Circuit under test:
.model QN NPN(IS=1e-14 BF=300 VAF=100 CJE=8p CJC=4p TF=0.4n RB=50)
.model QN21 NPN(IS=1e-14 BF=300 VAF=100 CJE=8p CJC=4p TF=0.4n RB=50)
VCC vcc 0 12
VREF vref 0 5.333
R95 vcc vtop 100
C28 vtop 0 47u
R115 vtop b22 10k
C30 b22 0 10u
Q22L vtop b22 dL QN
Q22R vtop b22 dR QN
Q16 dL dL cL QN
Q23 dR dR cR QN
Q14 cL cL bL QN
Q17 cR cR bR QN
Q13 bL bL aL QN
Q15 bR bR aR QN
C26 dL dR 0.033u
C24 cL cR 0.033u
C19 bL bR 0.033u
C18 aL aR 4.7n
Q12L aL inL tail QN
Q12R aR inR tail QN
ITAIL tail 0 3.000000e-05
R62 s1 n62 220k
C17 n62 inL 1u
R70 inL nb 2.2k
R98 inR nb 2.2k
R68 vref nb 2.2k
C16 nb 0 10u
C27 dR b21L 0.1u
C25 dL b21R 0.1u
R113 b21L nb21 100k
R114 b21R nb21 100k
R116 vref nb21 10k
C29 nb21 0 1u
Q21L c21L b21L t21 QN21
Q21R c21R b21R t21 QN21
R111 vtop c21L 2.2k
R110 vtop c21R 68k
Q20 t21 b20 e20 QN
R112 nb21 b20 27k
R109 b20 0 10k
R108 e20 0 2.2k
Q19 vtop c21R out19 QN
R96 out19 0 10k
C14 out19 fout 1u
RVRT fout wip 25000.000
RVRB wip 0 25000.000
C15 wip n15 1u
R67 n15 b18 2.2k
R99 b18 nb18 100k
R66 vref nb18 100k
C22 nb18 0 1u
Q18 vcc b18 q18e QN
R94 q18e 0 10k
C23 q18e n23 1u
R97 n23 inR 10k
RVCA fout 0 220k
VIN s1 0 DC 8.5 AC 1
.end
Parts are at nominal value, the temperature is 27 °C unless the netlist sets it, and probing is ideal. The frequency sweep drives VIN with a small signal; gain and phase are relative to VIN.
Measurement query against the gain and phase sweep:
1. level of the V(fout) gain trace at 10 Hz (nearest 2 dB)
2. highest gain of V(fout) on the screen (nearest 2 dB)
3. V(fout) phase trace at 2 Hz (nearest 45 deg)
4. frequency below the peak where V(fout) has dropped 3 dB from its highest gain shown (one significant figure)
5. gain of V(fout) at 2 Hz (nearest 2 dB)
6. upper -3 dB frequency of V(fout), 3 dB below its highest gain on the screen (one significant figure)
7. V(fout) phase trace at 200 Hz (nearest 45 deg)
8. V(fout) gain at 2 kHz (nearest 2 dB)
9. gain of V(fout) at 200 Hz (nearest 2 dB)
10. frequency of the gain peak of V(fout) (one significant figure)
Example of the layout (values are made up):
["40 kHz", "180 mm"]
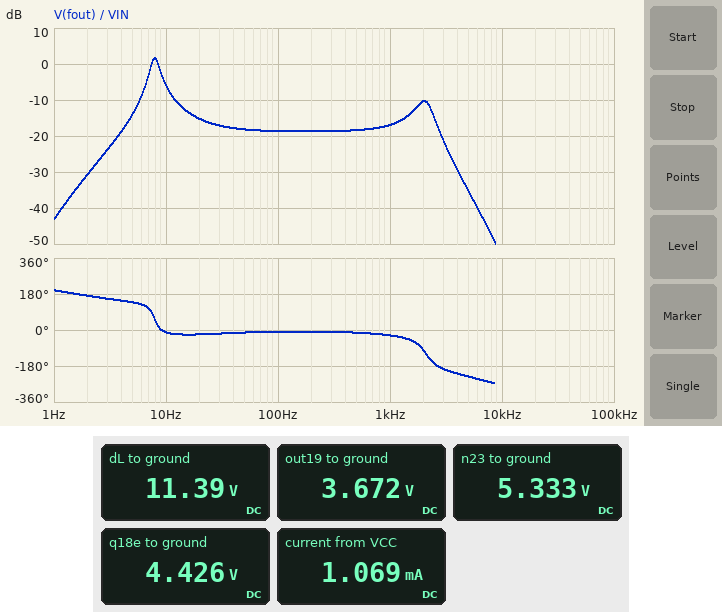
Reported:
["-6 dB", "2 dB", "180 deg", "7 Hz", "-30 dB", "9 Hz", "0 deg", "-10 dB", "-18 dB", "8 Hz"]
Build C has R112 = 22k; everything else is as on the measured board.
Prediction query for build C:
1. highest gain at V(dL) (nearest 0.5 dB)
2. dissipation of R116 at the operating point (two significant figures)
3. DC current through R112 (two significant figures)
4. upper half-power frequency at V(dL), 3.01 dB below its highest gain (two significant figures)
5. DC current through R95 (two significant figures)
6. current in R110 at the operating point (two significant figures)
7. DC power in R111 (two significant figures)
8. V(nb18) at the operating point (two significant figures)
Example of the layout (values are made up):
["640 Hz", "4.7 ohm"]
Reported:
["-45.0 dB", "160 µW", "130 µA", "70 Hz", "610 µA", "120 µA", "60 µW", "5.2 V"]
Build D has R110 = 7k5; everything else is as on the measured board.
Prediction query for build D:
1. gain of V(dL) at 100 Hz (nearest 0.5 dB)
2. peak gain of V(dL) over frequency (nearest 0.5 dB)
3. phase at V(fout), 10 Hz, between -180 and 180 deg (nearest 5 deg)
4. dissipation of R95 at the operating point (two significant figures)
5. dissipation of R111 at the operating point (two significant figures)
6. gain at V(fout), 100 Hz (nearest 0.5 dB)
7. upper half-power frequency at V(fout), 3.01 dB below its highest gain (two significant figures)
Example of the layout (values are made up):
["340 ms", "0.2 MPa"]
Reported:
["-53.5 dB", "-44.0 dB", "95 deg", "170 µW", "29 µW", "-23.5 dB", "550 Hz"]
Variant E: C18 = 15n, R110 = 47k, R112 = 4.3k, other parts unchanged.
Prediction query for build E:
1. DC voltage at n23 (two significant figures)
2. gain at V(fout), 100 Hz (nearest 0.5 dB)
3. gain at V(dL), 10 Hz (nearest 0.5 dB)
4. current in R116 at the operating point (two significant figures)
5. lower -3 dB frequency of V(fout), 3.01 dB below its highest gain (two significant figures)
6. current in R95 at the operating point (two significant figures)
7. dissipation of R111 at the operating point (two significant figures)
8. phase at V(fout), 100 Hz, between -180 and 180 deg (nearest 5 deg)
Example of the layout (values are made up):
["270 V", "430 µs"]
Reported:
["5.3 V", "-37.5 dB", "-45.5 dB", "220 µA", "110 Hz", "900 µA", "520 µW", "35 deg"]
